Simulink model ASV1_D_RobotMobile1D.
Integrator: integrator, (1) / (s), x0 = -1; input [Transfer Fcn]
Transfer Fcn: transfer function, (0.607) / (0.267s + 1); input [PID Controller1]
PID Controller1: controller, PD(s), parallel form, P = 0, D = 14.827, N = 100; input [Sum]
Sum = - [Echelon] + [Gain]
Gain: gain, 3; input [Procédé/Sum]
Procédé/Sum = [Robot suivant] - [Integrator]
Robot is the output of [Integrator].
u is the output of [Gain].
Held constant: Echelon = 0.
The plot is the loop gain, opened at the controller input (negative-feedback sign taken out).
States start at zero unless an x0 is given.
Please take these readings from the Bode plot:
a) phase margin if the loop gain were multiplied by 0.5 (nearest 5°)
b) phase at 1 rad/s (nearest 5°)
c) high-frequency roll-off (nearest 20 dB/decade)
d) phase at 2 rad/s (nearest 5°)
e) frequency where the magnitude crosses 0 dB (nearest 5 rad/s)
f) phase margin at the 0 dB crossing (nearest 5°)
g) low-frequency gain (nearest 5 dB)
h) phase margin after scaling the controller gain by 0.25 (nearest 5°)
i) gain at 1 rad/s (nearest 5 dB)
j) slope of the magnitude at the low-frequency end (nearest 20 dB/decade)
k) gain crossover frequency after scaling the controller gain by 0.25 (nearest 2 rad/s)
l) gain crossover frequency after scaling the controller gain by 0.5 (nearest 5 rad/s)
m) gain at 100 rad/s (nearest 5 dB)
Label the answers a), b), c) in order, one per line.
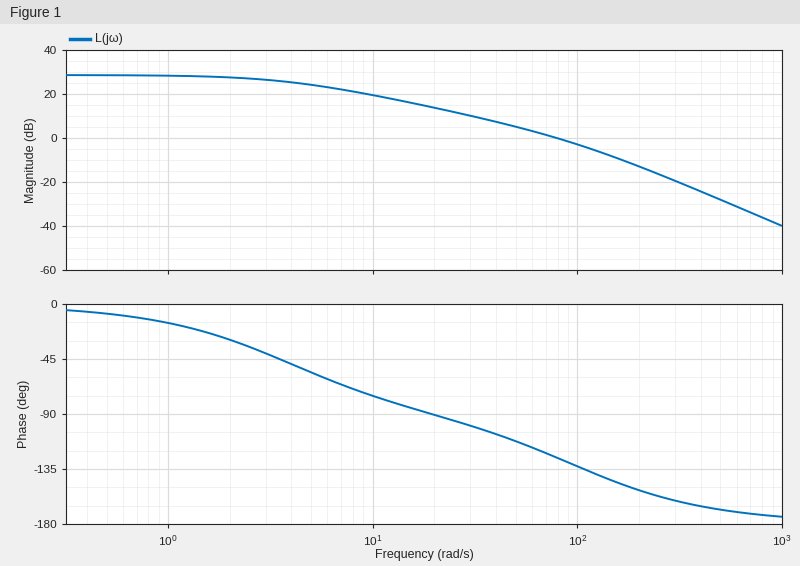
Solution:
a) 70°
b) -15°
c) -40 dB/decade
d) -30°
e) 80 rad/s
f) 55°
g) 30 dB
h) 85°
i) 30 dB
j) 0 dB/decade
k) 24 rad/s
l) 45 rad/s
m) -5 dB
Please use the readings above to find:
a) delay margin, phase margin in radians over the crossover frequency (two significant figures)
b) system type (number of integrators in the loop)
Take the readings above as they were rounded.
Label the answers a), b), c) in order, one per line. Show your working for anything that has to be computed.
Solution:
a) 55 × π / 180 / 80 = 0.012 s
b) 0
